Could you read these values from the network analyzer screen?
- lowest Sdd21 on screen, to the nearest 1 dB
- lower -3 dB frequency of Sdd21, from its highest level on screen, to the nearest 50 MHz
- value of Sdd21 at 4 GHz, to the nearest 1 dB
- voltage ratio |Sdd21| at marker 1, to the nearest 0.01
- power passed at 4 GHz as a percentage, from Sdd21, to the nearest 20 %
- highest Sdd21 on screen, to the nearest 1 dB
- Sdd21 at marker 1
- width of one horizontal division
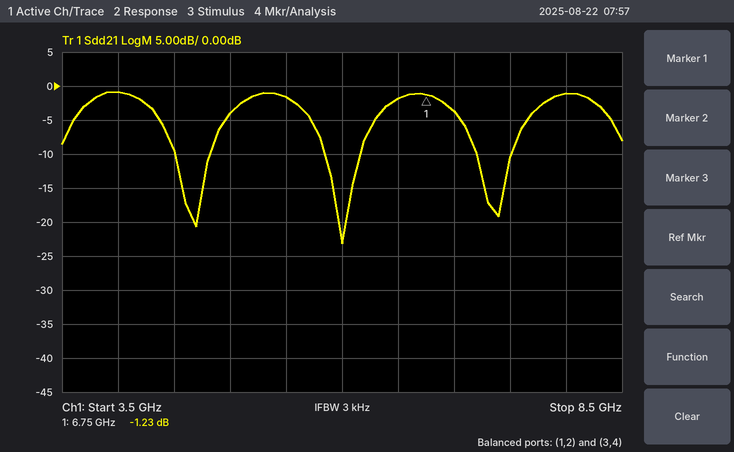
-23 dB
3.65 GHz
-1 dB
0.87
80 %
-1 dB
-1.23 dB
500 MHz
